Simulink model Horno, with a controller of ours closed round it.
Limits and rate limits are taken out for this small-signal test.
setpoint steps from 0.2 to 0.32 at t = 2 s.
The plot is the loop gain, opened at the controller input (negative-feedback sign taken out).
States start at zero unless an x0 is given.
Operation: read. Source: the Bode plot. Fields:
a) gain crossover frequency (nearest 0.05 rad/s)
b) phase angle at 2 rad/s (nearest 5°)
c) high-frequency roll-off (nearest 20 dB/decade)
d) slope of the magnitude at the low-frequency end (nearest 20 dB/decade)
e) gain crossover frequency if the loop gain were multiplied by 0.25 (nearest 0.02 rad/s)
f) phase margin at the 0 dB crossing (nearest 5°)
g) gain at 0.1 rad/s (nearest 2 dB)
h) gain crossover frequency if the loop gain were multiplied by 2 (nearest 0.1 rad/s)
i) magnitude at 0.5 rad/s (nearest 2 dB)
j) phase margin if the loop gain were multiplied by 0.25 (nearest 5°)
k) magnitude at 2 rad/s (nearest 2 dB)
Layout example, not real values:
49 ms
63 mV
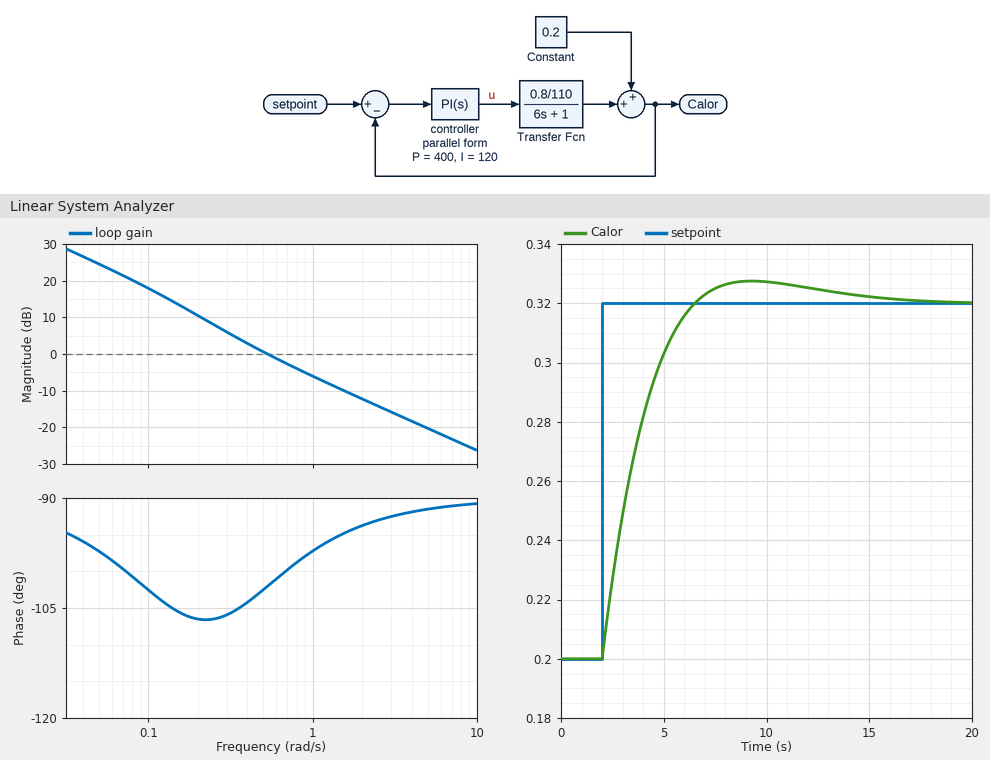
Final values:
0.55 rad/s
-95°
-20 dB/decade
-20 dB/decade
0.18 rad/s
80°
18 dB
1.0 rad/s
0 dB
75°
-12 dB
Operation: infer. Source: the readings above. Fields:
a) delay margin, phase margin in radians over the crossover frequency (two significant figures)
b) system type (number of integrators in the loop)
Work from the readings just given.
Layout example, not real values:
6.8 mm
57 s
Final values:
2.5 s
1
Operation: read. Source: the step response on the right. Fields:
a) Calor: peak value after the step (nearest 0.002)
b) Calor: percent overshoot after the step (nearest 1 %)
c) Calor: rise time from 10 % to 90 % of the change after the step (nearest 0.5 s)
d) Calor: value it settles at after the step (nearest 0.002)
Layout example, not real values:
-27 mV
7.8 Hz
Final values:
0.328
6 %
3.0 s
0.320
